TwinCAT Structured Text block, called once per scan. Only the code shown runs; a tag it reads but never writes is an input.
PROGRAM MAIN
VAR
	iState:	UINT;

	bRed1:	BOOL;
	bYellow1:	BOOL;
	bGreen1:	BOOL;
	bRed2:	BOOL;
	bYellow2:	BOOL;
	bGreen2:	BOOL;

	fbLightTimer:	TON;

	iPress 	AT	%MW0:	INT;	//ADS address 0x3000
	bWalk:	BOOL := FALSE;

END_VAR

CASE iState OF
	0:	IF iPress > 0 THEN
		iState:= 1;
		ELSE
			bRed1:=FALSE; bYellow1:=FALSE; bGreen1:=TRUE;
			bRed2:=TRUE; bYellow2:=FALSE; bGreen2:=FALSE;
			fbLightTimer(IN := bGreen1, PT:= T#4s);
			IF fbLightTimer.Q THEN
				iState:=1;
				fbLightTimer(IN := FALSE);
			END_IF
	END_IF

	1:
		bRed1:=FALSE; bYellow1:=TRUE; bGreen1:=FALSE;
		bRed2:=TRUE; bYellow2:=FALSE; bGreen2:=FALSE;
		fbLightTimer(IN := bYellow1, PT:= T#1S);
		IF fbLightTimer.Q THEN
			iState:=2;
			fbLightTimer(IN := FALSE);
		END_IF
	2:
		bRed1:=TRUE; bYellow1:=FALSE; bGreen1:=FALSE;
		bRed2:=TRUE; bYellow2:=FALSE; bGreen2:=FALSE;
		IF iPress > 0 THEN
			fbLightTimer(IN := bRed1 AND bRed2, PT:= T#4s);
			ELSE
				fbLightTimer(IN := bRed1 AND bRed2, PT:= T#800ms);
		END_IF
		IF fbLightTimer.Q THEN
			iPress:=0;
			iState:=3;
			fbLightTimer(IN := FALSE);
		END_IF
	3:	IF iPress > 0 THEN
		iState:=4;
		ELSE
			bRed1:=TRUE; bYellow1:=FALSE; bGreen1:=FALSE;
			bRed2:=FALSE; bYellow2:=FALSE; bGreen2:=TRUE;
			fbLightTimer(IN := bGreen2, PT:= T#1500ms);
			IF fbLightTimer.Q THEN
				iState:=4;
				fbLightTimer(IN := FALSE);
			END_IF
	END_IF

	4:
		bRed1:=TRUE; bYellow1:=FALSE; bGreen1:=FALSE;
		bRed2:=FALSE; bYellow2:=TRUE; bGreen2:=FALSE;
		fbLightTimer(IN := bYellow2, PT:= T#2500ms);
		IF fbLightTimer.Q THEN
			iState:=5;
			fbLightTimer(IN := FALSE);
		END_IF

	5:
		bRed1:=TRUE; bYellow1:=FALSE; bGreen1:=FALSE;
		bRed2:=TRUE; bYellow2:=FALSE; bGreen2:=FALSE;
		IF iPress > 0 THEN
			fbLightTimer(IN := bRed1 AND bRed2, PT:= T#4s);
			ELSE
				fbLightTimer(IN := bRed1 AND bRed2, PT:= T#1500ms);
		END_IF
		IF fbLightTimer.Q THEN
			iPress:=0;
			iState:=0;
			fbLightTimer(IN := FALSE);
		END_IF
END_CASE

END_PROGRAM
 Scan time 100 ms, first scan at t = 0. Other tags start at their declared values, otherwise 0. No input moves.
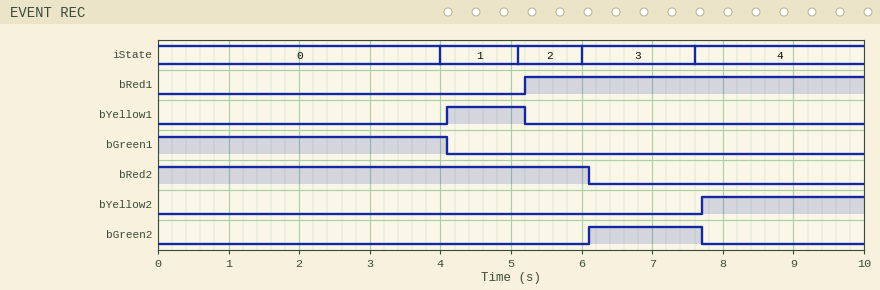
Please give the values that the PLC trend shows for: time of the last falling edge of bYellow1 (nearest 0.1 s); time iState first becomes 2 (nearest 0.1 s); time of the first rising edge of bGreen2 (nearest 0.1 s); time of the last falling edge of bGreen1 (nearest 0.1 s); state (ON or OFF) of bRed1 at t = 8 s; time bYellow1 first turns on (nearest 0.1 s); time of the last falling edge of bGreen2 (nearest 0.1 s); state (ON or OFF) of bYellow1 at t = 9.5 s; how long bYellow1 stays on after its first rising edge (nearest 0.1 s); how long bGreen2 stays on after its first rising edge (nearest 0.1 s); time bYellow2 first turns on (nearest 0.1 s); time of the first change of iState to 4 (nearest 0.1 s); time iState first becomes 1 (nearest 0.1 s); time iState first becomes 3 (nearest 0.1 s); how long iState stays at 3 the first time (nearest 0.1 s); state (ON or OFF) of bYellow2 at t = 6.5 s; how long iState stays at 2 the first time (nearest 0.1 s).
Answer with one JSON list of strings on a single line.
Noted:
["5.2 s", "5.1 s", "6.1 s", "4.1 s", "ON", "4.1 s", "7.7 s", "OFF", "1.1 s", "1.6 s", "7.7 s", "7.6 s", "4.0 s", "6.0 s", "1.6 s", "OFF", "0.9 s"]
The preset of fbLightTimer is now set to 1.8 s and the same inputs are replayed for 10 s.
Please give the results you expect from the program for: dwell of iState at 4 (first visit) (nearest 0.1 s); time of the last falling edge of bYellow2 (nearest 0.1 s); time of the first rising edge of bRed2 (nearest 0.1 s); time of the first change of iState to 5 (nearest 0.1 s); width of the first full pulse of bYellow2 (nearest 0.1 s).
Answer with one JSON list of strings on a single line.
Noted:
["1.9 s", "9.6 s", "9.6 s", "9.5 s", "1.9 s"]
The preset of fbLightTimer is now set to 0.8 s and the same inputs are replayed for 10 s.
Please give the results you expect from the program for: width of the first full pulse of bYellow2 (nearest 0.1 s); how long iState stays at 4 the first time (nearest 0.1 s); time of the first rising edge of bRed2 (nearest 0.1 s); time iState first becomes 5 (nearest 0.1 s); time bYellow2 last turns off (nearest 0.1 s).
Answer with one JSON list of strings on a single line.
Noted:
["0.9 s", "0.9 s", "8.6 s", "8.5 s", "8.6 s"]
